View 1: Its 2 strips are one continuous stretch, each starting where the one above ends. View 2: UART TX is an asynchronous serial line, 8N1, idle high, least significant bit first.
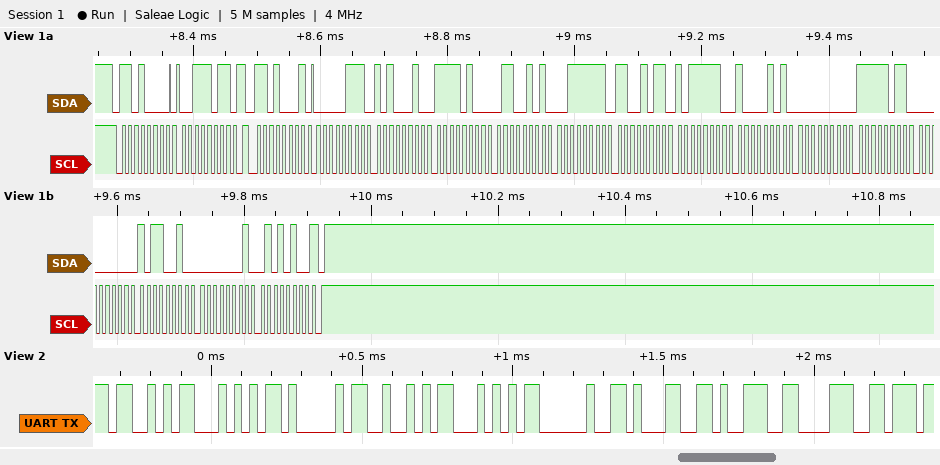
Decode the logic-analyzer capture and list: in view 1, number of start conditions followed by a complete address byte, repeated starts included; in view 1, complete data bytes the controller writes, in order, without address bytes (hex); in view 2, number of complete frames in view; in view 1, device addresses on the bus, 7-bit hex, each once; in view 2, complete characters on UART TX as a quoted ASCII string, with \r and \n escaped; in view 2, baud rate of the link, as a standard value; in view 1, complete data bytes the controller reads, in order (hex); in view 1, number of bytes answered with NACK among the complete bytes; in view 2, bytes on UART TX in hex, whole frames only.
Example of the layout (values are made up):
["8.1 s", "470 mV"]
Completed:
["2", "3B", "9", "0x68", "\"START 198\"", "38400 baud", "07 A2 F4 65 3F CB BE 85 00 FB 00 B2 01 54", "1", "53 54 41 52 54 20 31 39 38"]
